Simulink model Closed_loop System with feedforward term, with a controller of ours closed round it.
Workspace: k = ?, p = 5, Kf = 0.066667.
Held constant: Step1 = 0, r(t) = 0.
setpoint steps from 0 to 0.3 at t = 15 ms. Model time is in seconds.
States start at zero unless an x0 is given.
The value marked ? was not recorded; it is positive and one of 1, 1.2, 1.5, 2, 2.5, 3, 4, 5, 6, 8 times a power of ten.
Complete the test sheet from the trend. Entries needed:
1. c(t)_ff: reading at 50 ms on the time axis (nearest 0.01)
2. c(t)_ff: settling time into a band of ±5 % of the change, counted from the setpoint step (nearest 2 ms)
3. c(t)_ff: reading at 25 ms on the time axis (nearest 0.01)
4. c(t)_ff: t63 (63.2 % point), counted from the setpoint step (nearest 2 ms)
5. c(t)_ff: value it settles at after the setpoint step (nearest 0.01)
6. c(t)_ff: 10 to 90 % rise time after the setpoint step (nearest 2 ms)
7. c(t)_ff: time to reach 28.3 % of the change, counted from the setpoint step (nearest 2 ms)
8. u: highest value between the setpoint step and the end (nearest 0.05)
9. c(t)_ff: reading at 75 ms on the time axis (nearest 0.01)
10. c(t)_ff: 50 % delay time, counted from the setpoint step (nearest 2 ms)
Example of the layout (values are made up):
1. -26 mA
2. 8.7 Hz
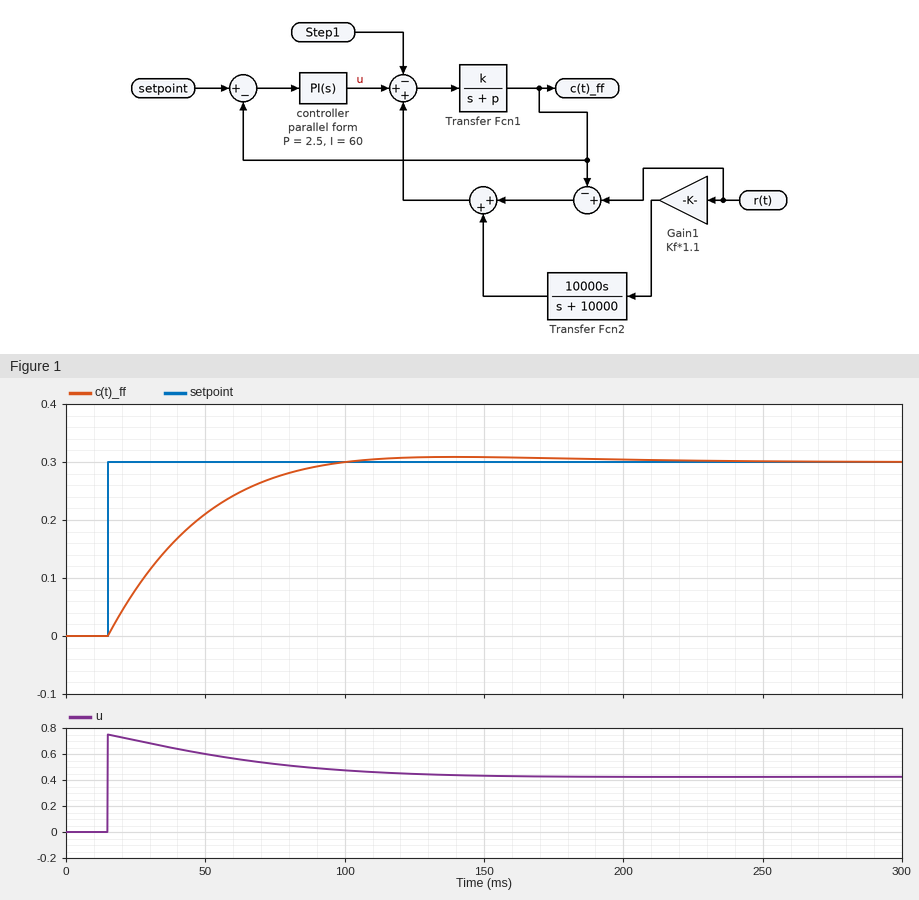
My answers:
1. 0.21
2. 68 ms
3. 0.08
4. 30 ms
5. 0.30
6. 54 ms
7. 10 ms
8. 0.75
9. 0.27
10. 22 ms
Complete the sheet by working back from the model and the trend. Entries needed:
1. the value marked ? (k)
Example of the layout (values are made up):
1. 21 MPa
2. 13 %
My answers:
1. 12
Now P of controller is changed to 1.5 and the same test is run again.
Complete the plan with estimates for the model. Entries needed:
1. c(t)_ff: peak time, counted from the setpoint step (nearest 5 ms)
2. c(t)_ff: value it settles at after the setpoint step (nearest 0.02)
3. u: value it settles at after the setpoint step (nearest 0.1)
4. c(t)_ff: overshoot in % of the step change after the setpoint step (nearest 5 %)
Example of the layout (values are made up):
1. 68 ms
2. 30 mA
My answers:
1. 120 ms
2. 0.30
3. 0.4
4. 10 %
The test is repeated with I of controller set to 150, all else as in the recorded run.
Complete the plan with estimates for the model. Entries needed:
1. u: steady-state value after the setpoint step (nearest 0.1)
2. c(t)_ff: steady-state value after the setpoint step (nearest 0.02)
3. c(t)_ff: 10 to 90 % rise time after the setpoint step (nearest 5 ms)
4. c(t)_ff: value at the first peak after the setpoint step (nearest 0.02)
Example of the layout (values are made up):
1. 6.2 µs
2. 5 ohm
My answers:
1. 0.4
2. 0.30
3. 30 ms
4. 0.36
